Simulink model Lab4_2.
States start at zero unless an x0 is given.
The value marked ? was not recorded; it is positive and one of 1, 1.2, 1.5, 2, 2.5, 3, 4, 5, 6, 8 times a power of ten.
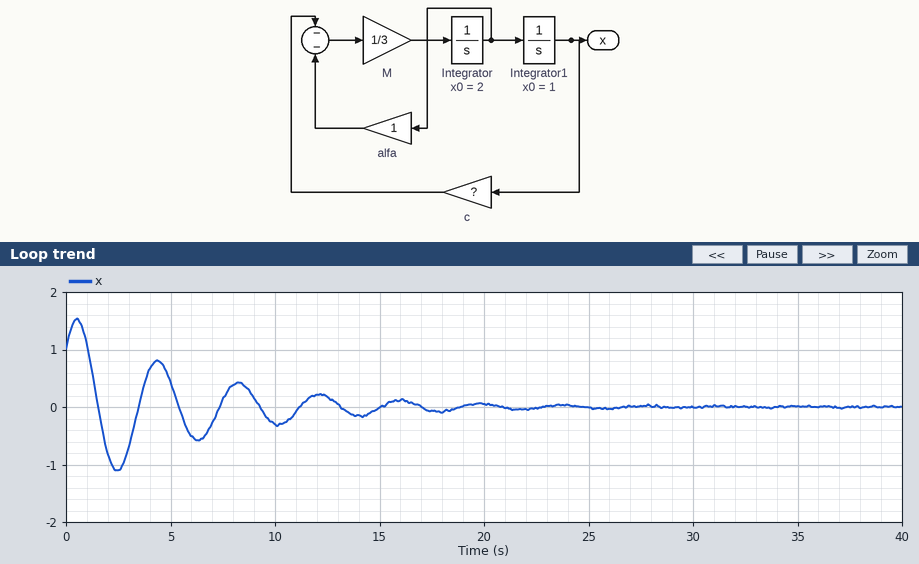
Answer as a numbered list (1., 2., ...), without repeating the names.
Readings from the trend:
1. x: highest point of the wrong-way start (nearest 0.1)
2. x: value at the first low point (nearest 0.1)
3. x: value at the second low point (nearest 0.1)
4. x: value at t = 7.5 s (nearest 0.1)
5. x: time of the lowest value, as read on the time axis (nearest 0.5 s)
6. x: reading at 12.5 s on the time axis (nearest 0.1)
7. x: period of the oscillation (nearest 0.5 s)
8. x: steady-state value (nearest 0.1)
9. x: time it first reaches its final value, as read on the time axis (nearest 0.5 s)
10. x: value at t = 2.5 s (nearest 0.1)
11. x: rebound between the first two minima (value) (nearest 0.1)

1. 1.5
2. -1.1
3. -0.6
4. 0.1
5. 2.5 s
6. 0.2
7. 4.0 s
8. 0.0
9. 1.5 s
10. -1.1
11. 0.8
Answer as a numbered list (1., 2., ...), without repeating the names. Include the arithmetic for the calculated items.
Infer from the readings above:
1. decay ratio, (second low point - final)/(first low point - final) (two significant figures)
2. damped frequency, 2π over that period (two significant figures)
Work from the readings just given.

1. (-0.6 - 0) / (-1.1 - 0) = 0.55
2. 2π / 4 = 1.6 rad/s
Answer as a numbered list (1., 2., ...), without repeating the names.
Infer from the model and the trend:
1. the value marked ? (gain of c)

1. 8
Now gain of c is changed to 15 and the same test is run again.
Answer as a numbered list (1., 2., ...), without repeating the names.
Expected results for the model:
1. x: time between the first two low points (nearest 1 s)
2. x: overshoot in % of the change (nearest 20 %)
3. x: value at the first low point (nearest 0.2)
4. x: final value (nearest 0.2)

1. 3 s
2. 100 %
3. -1.0
4. 0.0
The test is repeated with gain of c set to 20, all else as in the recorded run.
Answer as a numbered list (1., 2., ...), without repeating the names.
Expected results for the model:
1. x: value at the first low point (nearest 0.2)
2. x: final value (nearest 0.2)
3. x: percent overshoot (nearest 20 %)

1. -1.0
2. 0.0
3. 100 %
